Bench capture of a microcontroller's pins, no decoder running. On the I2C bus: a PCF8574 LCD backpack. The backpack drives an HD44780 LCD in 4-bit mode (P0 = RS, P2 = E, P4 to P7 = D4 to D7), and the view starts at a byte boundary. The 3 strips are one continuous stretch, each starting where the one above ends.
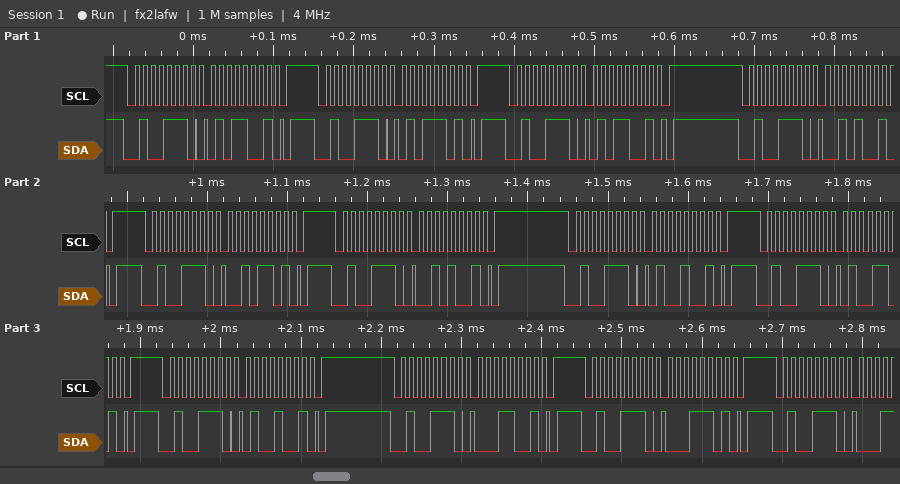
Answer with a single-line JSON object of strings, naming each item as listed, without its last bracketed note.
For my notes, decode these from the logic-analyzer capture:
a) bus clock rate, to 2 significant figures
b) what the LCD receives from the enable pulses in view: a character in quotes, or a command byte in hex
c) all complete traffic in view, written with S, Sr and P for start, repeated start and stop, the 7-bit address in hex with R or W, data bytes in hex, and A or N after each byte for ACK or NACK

{"bus clock rate, to 2 significant figures": "100 kHz", "what the LCD receives from the enable pulses in view: a character in quotes, or a command byte in hex": "'R'", "all complete traffic in view, written with S, Sr and P for start, repeated start and stop, the 7-bit address in hex with R or W, data bytes in hex, and A or N after each byte for ACK or NACK": "S 27W A 59 A P S 27W A 5D A P S 27W A 59 A P S 27W A 29 A P S 27W A 2D A P S 27W A 29 A P S 27W A 49 A P S 27W A 4D A P S 27W A 49 A P S 27W A 19 A P S 27W A 1D A P S 27W A"}
